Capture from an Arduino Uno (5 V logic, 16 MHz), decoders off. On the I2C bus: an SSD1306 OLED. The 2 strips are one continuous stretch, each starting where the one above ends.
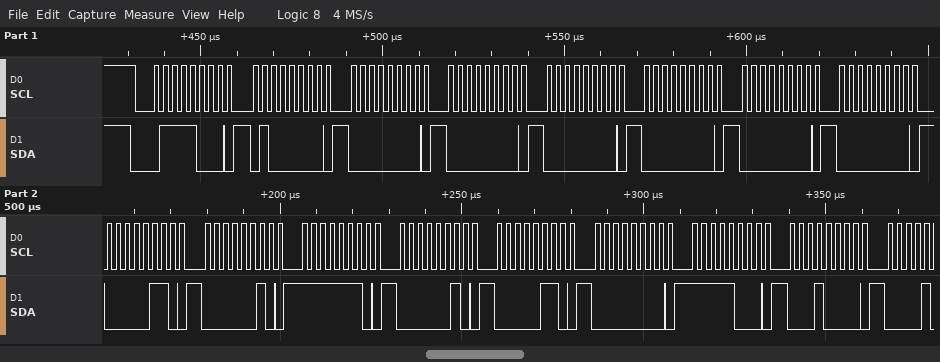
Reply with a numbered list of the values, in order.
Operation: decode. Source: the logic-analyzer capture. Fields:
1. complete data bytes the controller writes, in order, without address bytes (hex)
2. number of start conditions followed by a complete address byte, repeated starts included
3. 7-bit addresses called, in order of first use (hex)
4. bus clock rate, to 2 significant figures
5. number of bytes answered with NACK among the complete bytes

1. 40 00 00 00 00 00 00 06 02 FE 02 06 00 F8 10
2. 1
3. 0x3C
4. 400 kHz
5. 0
